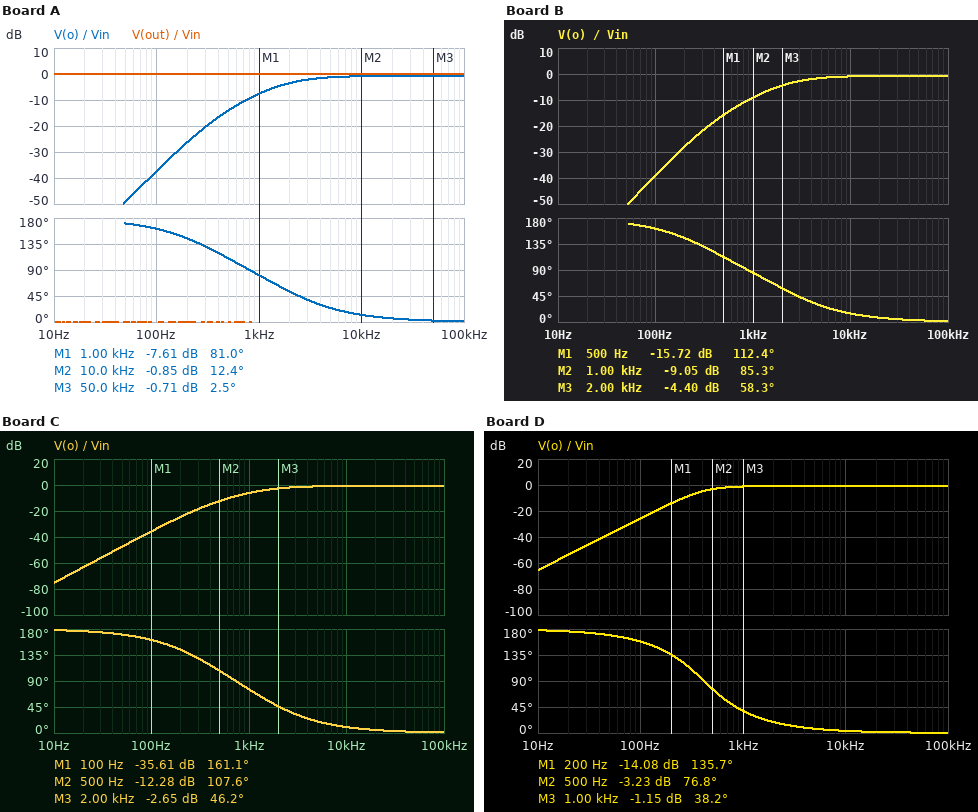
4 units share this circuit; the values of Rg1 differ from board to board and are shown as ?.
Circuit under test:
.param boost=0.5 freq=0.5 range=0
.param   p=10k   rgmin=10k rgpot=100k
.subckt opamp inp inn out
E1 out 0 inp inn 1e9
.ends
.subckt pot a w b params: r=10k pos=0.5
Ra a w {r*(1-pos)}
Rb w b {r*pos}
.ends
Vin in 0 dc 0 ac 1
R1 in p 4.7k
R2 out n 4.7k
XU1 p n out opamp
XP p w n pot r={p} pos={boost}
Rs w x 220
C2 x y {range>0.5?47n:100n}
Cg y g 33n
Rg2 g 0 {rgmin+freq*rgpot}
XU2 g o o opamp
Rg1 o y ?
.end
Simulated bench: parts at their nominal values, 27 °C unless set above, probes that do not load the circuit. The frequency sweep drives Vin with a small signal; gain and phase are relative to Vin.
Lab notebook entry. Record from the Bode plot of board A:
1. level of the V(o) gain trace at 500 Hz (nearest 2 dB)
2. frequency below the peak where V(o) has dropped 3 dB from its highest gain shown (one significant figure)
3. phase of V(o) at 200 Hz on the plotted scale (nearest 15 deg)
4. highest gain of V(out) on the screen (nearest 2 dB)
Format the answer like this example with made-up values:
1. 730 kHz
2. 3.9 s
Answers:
1. -14 dB
2. 2 kHz
3. 150 deg
4. 0 dB
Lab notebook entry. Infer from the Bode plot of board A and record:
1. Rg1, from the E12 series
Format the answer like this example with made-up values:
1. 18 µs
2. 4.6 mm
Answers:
1. 180 Ω
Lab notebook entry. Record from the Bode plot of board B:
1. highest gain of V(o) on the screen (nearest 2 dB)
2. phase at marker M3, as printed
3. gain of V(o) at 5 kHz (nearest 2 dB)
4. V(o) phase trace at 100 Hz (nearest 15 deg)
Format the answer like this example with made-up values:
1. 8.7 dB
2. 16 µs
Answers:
1. 0 dB
2. 58.3 deg
3. -2 dB
4. 165 deg
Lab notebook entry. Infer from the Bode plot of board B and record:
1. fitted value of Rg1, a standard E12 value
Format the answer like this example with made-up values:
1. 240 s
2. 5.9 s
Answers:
1. 150 Ω
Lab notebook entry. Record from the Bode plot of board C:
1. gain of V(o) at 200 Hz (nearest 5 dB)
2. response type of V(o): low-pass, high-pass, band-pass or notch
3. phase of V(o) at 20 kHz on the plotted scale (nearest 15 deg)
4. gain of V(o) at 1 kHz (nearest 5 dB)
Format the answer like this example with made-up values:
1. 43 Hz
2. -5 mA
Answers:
1. -25 dB
2. high-pass
3. 0 deg
4. -5 dB
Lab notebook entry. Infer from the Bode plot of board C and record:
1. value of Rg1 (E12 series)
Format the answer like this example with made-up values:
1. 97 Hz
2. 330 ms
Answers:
1. 220 Ω
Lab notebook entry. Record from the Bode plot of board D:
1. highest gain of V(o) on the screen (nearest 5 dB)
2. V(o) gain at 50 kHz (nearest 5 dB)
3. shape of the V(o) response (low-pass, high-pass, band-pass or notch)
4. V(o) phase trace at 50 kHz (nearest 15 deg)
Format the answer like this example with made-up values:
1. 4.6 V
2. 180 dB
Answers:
1. 0 dB
2. 0 dB
3. high-pass
4. 0 deg
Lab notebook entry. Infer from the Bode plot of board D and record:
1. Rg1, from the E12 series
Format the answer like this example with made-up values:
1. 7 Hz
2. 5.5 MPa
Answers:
1. 680 Ω
